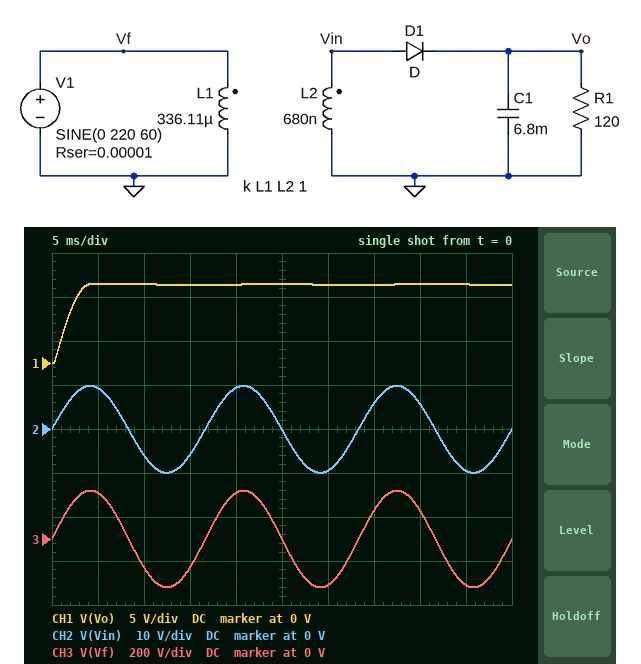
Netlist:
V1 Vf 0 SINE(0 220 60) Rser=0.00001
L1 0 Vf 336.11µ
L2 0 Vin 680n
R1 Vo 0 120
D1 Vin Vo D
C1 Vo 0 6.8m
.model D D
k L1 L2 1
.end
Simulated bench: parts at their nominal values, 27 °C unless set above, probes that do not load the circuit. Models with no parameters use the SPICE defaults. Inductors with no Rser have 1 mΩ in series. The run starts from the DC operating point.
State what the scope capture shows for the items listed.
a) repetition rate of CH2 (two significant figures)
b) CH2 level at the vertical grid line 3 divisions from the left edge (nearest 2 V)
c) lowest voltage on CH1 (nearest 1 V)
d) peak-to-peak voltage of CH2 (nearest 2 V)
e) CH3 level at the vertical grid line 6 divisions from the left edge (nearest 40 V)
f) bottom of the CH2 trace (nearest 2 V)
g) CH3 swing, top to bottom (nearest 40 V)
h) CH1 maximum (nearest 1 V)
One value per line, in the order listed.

60 Hz
-6 V
0 V
20 V
-200 V
-10 V
440 V
9 V
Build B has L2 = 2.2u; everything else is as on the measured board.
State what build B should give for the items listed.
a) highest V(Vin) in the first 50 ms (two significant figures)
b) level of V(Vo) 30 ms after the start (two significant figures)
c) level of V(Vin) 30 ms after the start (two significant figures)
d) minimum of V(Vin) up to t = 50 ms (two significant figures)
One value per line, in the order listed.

18 V
17 V
-17 V
-18 V
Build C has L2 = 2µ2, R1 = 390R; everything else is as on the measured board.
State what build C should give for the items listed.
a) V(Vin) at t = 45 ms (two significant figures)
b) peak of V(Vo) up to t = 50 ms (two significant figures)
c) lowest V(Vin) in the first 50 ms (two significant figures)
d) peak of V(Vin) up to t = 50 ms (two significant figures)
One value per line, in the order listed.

-17 V
17 V
-18 V
18 V
